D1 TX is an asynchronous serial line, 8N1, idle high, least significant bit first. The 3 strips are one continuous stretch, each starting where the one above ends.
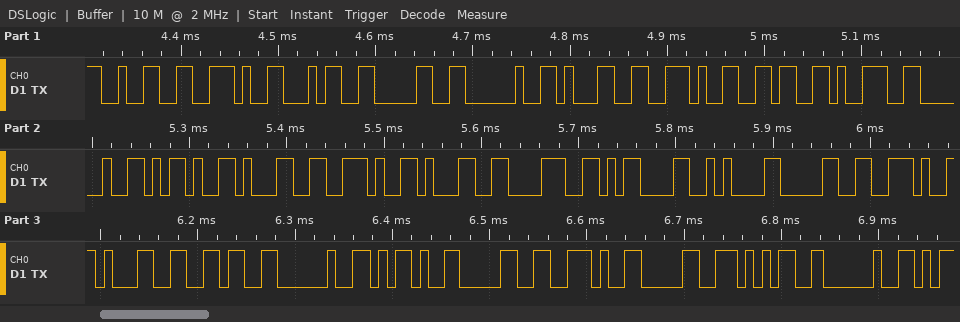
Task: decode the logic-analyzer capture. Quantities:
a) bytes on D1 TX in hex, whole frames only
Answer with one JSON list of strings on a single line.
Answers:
["32 2E 34 30 20 31 2E 36 39 20 2D 31 2E 31 38 0D 0A 30 2E 31 36 20 2D 30 2E 30 35 20"]
